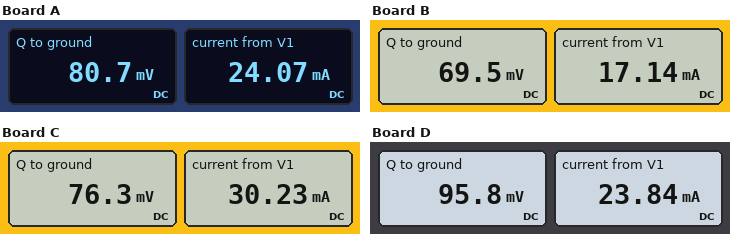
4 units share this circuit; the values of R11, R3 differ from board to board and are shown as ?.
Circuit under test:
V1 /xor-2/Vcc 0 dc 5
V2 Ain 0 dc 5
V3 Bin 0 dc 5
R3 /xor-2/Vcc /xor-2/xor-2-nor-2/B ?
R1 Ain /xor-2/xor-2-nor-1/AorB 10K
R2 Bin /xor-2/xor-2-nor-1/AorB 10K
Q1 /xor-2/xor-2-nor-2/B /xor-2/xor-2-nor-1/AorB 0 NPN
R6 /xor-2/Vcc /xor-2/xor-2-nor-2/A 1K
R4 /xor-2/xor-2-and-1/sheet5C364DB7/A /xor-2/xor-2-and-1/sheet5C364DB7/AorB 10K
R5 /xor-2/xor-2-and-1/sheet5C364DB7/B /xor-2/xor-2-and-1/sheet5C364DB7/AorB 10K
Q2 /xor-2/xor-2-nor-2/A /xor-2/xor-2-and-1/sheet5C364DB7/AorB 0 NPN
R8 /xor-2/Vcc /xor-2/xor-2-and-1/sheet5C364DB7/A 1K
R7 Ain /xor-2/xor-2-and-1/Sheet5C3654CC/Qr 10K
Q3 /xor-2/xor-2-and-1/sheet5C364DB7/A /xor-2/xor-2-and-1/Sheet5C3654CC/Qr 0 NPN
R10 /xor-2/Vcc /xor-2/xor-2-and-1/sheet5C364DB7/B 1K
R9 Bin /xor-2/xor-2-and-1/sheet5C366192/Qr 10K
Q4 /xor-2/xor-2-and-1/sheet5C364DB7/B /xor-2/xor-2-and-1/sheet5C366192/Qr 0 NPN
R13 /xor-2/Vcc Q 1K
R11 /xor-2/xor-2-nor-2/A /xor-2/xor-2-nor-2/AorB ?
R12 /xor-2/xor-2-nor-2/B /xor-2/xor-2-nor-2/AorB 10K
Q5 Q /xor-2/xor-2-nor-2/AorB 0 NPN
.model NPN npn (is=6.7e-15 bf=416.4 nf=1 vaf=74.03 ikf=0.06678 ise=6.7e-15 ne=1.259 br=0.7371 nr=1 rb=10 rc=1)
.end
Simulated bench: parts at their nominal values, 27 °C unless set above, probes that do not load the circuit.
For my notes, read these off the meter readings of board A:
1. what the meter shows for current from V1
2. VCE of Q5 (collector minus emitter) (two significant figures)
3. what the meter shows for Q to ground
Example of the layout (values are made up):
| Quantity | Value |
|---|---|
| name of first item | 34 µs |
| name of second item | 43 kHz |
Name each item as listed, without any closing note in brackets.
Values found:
| Quantity | Value |
|---|---|
| what the meter shows for current from V1 | 24.07 mA |
| VCE of Q5 (collector minus emitter) | 81 mV |
| what the meter shows for Q to ground | 80.7 mV |
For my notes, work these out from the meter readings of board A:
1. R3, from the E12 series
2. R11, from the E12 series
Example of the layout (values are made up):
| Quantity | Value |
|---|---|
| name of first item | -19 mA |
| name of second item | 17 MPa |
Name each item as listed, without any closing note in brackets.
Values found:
| Quantity | Value |
|---|---|
| R3, from the E12 series | 560 Ω |
| R11, from the E12 series | 6.8 kΩ |
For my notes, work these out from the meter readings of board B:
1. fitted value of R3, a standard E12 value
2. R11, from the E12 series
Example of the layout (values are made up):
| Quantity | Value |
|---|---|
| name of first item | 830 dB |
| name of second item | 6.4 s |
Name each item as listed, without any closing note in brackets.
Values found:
| Quantity | Value |
|---|---|
| fitted value of R3, a standard E12 value | 3.3 kΩ |
| R11, from the E12 series | 3.9 kΩ |
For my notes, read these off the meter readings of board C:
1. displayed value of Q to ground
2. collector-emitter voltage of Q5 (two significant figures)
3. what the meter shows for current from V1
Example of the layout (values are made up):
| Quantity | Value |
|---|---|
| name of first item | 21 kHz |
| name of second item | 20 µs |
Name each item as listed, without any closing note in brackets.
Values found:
| Quantity | Value |
|---|---|
| displayed value of Q to ground | 76.3 mV |
| collector-emitter voltage of Q5 | 76 mV |
| what the meter shows for current from V1 | 30.23 mA |
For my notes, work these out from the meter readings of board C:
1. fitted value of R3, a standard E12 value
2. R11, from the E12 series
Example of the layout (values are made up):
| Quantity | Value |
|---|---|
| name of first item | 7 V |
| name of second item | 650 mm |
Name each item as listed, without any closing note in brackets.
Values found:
| Quantity | Value |
|---|---|
| fitted value of R3, a standard E12 value | 330 Ω |
| R11, from the E12 series | 5.6 kΩ |
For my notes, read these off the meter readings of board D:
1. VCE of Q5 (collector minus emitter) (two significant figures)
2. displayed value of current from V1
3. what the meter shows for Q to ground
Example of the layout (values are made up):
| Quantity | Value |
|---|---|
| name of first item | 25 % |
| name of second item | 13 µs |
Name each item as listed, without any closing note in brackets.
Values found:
| Quantity | Value |
|---|---|
| VCE of Q5 (collector minus emitter) | 96 mV |
| displayed value of current from V1 | 23.84 mA |
| what the meter shows for Q to ground | 95.8 mV |
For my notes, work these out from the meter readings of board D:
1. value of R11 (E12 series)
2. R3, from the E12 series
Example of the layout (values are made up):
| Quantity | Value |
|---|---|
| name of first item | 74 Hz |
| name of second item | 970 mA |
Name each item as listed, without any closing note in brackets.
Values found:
| Quantity | Value |
|---|---|
| value of R11 | 12 kΩ |
| R3, from the E12 series | 560 Ω |
